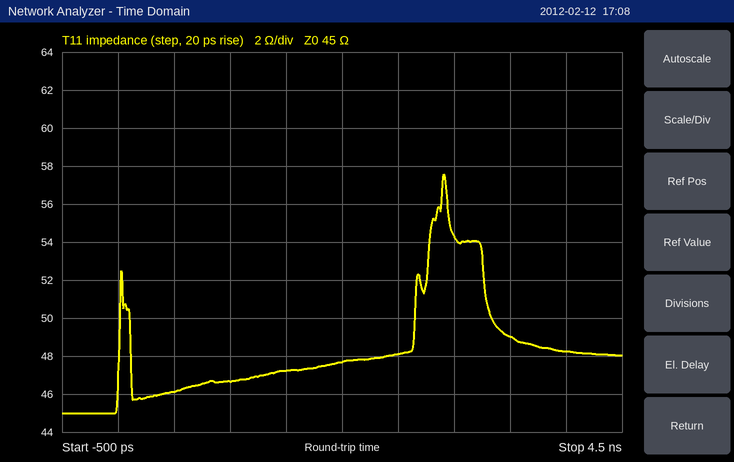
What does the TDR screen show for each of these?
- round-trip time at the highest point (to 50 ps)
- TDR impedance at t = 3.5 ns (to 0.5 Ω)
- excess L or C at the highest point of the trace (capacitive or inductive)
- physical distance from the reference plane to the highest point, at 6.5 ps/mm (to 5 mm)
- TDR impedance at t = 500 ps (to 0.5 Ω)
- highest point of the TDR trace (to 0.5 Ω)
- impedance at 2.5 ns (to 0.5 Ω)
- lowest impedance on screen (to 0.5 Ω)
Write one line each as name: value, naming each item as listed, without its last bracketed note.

round-trip time at the highest point: 2.90 ns
TDR impedance at t = 3.5 ns: 49.0 Ω
excess L or C at the highest point of the trace: inductive
physical distance from the reference plane to the highest point, at 6.5 ps/mm: 225 mm
TDR impedance at t = 500 ps: 46.0 Ω
highest point of the TDR trace: 57.5 Ω
impedance at 2.5 ns: 48.0 Ω
lowest impedance on screen: 45.0 Ω
